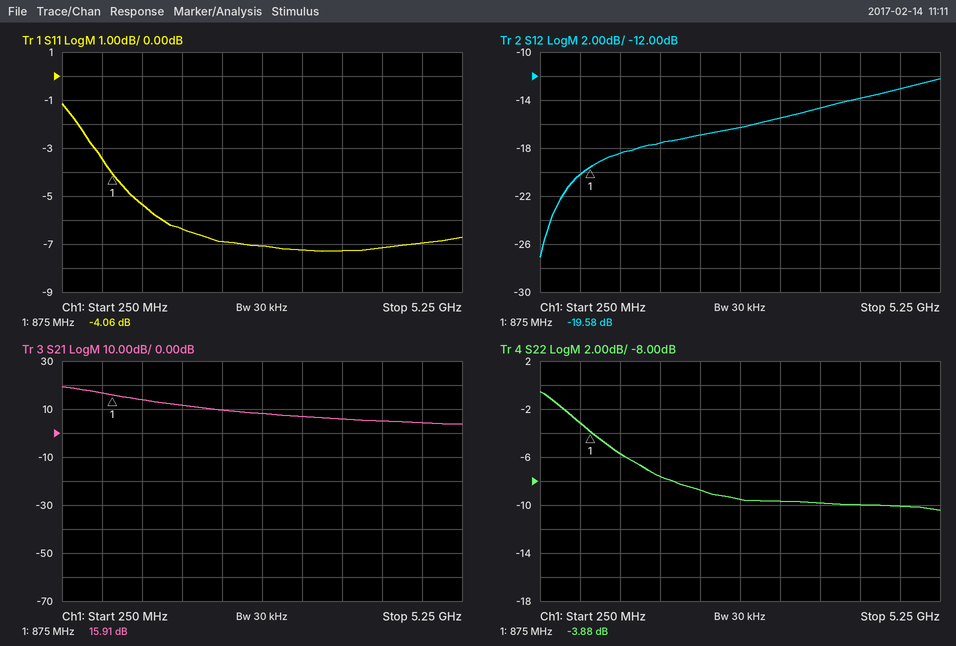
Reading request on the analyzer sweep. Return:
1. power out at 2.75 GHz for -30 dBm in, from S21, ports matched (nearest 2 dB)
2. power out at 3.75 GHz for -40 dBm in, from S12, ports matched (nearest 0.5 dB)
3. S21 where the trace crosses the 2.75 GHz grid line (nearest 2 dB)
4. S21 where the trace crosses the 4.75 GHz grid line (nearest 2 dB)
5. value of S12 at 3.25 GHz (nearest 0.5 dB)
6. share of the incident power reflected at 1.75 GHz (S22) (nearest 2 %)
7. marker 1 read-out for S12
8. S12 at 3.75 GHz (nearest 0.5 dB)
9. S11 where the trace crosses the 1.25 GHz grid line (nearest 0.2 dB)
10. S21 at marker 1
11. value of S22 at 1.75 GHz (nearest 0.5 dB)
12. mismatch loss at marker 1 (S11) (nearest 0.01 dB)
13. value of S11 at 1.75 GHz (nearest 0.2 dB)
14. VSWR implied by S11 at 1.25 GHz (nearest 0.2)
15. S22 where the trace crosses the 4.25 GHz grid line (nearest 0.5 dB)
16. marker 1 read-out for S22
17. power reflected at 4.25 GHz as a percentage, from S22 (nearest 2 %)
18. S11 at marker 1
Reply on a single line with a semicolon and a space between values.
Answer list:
-22 dBm; -54.5 dBm; 8 dB; 4 dB; -15.5 dB; 18 %; -19.58 dB; -14.5 dB; -5.4 dB; 15.91 dB; -7.5 dB; 2.17 dB; -6.4 dB; 3.4; -10.0 dB; -3.88 dB; 10 %; -4.06 dB
